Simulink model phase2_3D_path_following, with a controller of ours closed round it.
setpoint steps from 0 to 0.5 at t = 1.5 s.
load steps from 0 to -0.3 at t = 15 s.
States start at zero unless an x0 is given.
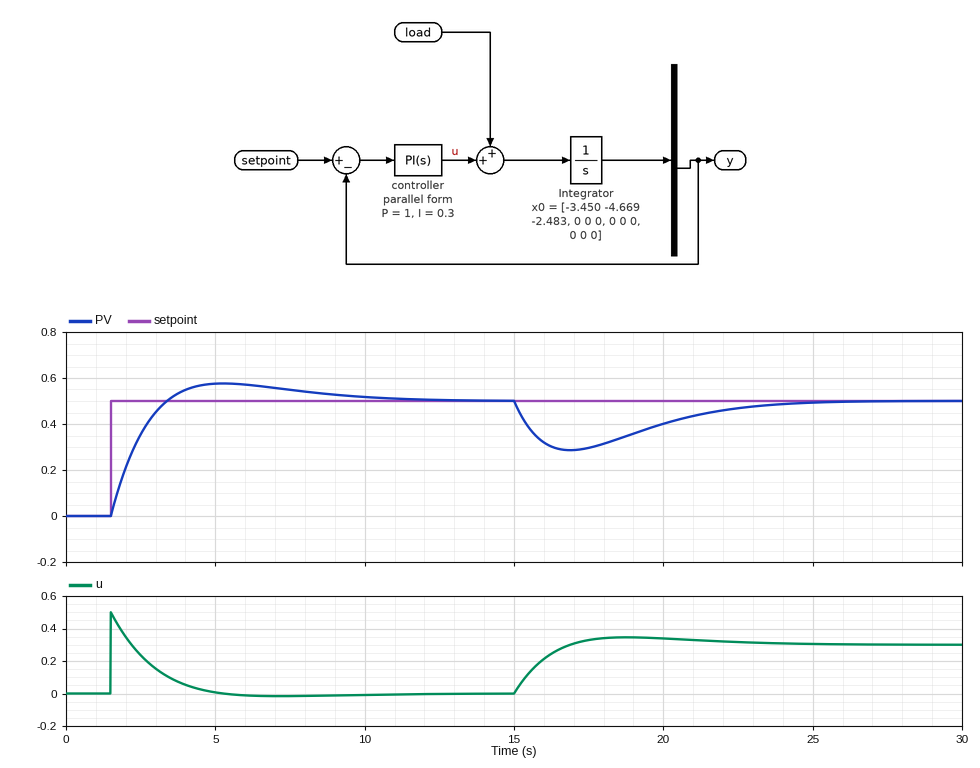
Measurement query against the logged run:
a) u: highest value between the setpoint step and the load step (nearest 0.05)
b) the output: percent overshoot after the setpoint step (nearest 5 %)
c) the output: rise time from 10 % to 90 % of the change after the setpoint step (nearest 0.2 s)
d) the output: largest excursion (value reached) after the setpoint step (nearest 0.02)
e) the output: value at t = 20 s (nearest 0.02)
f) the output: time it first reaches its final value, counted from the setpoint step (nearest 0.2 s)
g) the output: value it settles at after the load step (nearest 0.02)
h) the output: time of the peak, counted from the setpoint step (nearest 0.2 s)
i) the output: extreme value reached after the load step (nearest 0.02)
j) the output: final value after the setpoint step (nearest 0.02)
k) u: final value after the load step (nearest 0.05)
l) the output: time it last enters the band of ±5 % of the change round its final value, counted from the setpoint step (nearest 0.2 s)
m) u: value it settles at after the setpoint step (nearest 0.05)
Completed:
0.50
15 %
1.4 s
0.58
0.40
1.8 s
0.50
3.8 s
0.28
0.50
0.30
7.8 s
0.00
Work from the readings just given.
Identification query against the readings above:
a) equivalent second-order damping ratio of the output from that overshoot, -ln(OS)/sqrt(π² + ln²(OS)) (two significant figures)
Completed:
0.52
